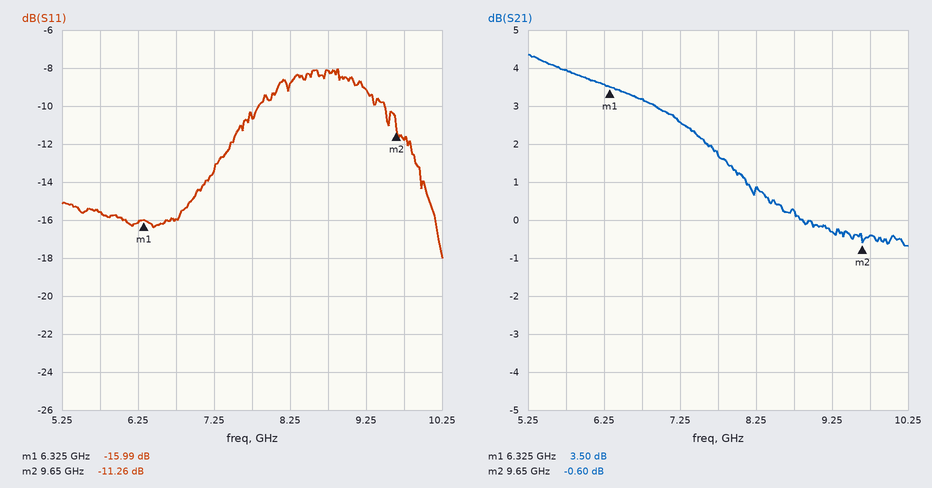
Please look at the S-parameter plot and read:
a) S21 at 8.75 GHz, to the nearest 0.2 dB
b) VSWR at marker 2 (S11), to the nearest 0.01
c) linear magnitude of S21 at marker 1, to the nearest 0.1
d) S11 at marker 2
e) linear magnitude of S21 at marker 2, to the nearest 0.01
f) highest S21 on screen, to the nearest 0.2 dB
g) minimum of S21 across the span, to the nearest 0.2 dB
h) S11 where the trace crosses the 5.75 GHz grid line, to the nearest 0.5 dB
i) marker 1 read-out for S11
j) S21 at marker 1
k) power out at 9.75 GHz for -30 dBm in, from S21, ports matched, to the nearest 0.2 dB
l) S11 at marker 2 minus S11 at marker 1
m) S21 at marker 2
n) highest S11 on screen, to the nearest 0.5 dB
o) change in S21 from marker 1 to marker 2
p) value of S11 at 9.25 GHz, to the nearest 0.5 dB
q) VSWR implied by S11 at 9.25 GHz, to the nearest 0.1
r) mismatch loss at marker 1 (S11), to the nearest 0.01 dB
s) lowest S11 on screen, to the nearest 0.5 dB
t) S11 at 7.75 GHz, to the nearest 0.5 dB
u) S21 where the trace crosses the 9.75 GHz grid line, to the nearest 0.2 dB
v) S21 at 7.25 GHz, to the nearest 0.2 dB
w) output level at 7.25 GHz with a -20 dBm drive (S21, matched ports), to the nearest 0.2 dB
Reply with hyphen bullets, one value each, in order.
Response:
- 0.2 dB
- 1.75
- 1.5
- -11.26 dB
- 0.93
- 4.4 dB
- -0.6 dB
- -15.5 dB
- -15.99 dB
- 3.50 dB
- -30.4 dBm
- 4.73 dB
- -0.60 dB
- -8.0 dB
- -4.10 dB
- -9.0 dB
- 2.1
- 0.11 dB
- -18.0 dB
- -10.5 dB
- -0.4 dB
- 2.6 dB
- -17.4 dBm
